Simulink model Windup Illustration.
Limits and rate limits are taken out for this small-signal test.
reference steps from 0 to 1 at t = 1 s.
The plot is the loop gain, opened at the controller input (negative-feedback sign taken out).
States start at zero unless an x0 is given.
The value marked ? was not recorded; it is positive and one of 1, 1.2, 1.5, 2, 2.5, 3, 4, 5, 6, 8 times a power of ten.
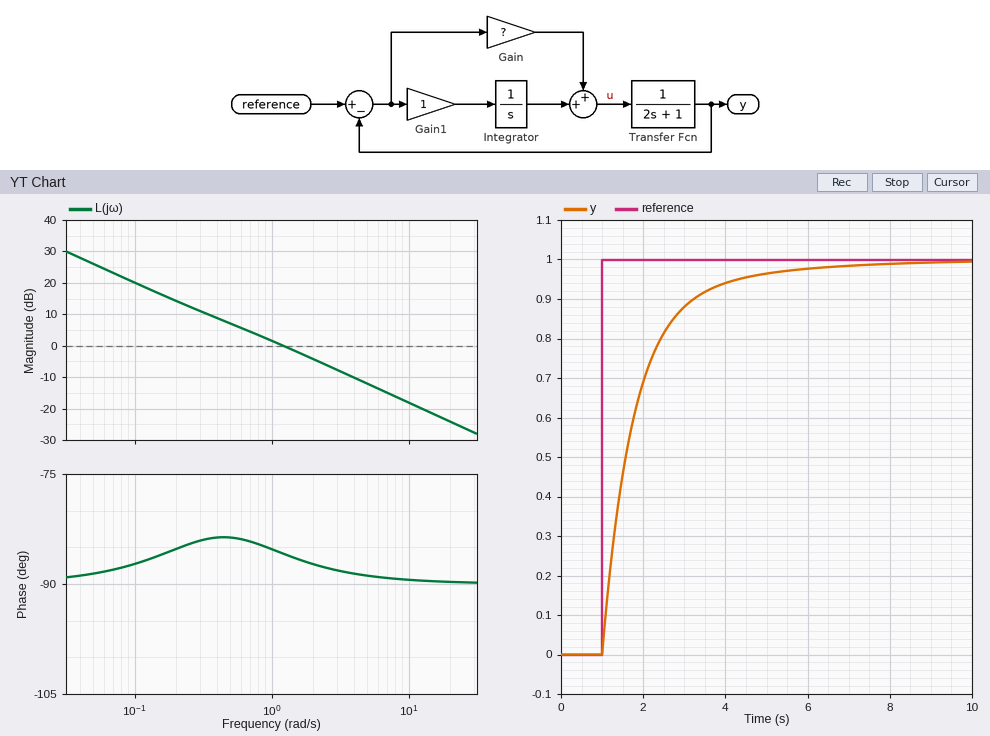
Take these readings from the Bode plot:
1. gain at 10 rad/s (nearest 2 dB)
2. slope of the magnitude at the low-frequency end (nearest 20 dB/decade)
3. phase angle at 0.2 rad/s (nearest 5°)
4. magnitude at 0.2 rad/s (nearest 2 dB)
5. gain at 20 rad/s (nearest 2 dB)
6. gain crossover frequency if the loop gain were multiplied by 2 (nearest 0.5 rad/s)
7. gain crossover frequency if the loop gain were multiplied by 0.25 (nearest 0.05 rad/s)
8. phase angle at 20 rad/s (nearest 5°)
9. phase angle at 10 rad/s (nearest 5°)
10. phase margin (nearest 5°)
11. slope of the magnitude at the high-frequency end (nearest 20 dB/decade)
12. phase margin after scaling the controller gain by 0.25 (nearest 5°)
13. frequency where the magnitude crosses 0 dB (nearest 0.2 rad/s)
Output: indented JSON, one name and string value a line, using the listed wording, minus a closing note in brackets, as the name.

{
  "gain at 10 rad/s": "-18 dB",
  "slope of the magnitude at the low-frequency end": "-20 dB/decade",
  "phase angle at 0.2 rad/s": "-85°",
  "magnitude at 0.2 rad/s": "14 dB",
  "gain at 20 rad/s": "-24 dB",
  "gain crossover frequency if the loop gain were multiplied by 2": "2.5 rad/s",
  "gain crossover frequency if the loop gain were multiplied by 0.25": "0.25 rad/s",
  "phase angle at 20 rad/s": "-90°",
  "phase angle at 10 rad/s": "-90°",
  "phase margin": "95°",
  "slope of the magnitude at the high-frequency end": "-20 dB/decade",
  "phase margin after scaling the controller gain by 0.25": "95°",
  "frequency where the magnitude crosses 0 dB": "1.2 rad/s"
}
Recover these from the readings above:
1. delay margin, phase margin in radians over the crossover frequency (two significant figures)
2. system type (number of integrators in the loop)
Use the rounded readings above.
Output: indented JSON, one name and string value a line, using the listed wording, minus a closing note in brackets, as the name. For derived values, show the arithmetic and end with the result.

{
  "delay margin, phase margin in radians over the crossover frequency": "95 × π / 180 / 1.2 = 1.4 s",
  "system type": "1"
}
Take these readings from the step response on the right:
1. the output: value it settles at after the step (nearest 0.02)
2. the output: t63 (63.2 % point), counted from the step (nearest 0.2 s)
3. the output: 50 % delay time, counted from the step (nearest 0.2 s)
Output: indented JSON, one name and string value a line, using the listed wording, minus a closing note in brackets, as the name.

{
  "the output: value it settles at after the step": "1.00",
  "the output: t63 (63.2 % point), counted from the step": "0.8 s",
  "the output: 50 % delay time, counted from the step": "0.6 s"
}
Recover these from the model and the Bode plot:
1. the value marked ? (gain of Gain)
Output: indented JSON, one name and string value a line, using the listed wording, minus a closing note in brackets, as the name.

{
  "the value marked ?": "2.5"
}
